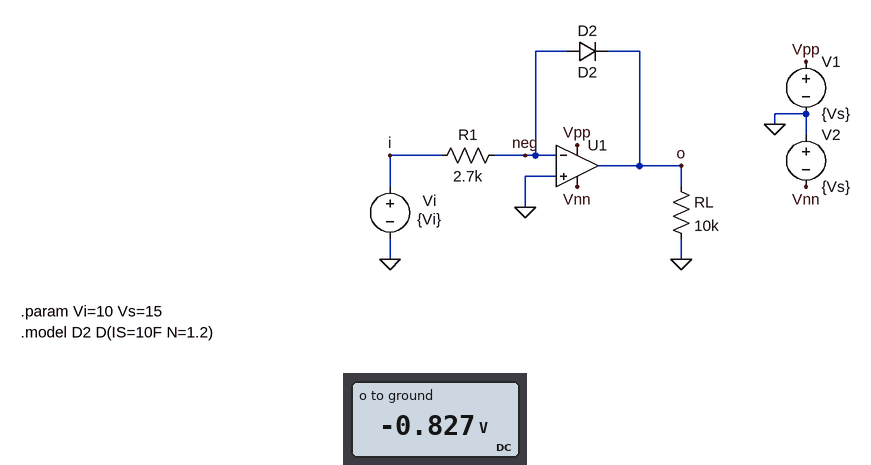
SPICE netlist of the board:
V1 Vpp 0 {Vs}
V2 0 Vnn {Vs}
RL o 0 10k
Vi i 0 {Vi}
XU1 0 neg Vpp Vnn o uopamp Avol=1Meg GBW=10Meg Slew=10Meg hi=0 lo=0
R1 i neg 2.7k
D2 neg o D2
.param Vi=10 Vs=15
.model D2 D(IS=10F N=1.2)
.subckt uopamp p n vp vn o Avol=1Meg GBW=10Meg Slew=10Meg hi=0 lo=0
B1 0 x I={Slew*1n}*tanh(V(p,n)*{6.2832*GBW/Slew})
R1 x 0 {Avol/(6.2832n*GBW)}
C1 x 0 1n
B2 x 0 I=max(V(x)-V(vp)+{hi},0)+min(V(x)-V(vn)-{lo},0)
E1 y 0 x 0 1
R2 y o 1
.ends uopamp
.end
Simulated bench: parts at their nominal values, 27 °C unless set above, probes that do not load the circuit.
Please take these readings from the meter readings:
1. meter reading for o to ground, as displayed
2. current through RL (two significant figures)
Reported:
-0.827 V
83 µA
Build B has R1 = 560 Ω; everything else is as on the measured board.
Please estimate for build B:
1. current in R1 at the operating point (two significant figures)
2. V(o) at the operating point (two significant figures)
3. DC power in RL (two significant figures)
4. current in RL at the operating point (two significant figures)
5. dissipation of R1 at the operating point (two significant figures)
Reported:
18 mA
-880 mV
77 µW
88 µA
180 mW
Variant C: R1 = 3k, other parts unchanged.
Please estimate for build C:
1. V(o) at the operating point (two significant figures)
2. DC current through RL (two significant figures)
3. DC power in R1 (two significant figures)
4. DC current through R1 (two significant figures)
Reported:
-820 mV
82 µA
33 mW
3.3 mA
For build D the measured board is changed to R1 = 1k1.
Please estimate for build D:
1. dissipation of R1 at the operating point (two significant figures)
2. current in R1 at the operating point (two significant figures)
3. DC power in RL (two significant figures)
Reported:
91 mW
9.1 mA
73 µW
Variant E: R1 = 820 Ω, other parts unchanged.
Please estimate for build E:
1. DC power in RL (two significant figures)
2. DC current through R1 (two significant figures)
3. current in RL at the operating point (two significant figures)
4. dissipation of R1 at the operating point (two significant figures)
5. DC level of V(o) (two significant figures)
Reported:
75 µW
12 mA
86 µA
120 mW
-860 mV
